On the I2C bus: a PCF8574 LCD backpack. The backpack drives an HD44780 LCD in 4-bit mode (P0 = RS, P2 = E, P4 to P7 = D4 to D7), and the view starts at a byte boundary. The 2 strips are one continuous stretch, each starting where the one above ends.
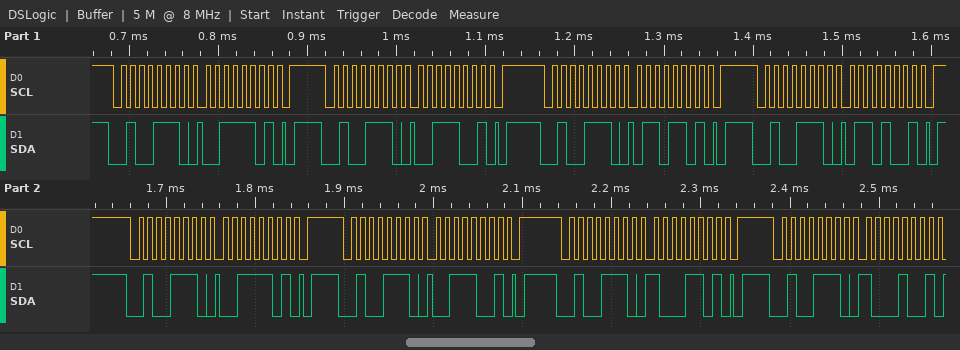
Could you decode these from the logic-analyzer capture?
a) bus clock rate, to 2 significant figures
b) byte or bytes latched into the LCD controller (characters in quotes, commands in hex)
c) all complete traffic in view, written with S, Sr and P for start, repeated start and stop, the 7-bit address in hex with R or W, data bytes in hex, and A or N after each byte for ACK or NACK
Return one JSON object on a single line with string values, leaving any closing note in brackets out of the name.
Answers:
{"bus clock rate, to 2 significant figures": "100 kHz", "byte or bytes latched into the LCD controller": "'6' '8'", "all complete traffic in view, written with S, Sr and P for start, repeated start and stop, the 7-bit address in hex with R or W, data bytes in hex, and A or N after each byte for ACK or NACK": "S 27W A 3D A P S 27W A 39 A P S 27W A 6D A P S 27W A 69 A P S 27W A 3D A P S 27W A 39 A P S 27W A 8D A P S 27W A 89 A"}
